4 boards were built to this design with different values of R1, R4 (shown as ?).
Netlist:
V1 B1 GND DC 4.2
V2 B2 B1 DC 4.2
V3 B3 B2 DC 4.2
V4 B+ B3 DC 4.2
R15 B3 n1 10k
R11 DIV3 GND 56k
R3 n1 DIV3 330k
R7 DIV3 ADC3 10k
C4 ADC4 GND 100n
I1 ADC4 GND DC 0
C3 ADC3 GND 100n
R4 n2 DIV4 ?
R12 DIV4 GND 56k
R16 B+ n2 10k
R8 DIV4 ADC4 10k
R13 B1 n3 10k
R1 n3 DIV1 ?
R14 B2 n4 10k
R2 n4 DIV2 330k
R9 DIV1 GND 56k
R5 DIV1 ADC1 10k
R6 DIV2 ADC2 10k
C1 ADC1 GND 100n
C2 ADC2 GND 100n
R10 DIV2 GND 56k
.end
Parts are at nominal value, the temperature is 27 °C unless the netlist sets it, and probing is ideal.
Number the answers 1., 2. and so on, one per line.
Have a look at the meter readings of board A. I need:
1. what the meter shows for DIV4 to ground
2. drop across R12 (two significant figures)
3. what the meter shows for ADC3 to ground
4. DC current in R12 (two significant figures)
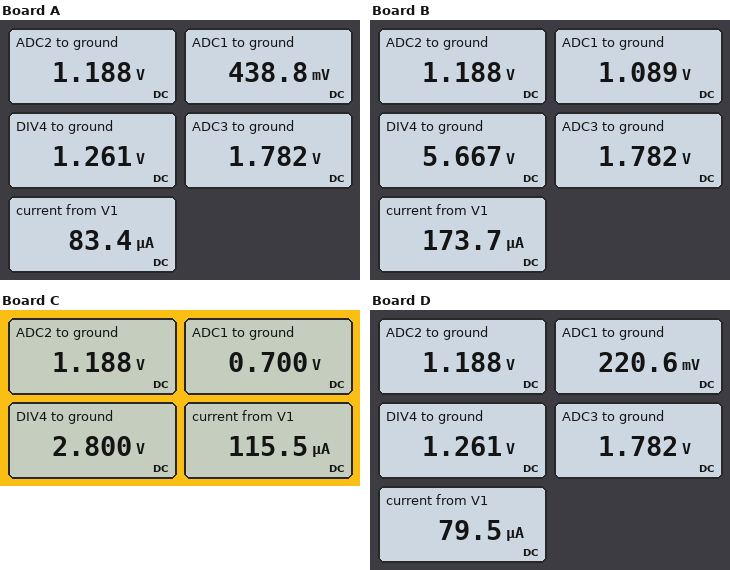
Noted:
1. 1.261 V
2. 1.3 V
3. 1.782 V
4. 23 µA
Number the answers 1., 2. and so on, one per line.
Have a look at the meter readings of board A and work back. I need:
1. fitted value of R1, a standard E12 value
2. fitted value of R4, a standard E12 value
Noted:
1. 470 kΩ
2. 680 kΩ
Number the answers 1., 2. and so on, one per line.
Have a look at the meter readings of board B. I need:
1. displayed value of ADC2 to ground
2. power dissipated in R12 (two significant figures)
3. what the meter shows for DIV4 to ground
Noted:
1. 1.188 V
2. 570 µW
3. 5.667 V
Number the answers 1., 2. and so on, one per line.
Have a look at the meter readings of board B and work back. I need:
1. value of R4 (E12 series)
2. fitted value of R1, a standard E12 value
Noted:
1. 100 kΩ
2. 150 kΩ
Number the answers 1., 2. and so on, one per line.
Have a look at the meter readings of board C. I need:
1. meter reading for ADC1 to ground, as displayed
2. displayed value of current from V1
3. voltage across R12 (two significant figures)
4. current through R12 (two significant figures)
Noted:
1. 0.700 V
2. 115.5 µA
3. 2.8 V
4. 50 µA
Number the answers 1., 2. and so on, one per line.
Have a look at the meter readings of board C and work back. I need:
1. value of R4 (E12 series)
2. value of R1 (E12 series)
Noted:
1. 270 kΩ
2. 270 kΩ
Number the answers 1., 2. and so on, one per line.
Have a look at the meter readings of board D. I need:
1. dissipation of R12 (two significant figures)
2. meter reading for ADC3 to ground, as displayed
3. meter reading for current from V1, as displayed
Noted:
1. 28 µW
2. 1.782 V
3. 79.5 µA
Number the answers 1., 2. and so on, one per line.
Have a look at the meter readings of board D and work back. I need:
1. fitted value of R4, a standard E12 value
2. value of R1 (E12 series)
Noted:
1. 680 kΩ
2. 1 MΩ
